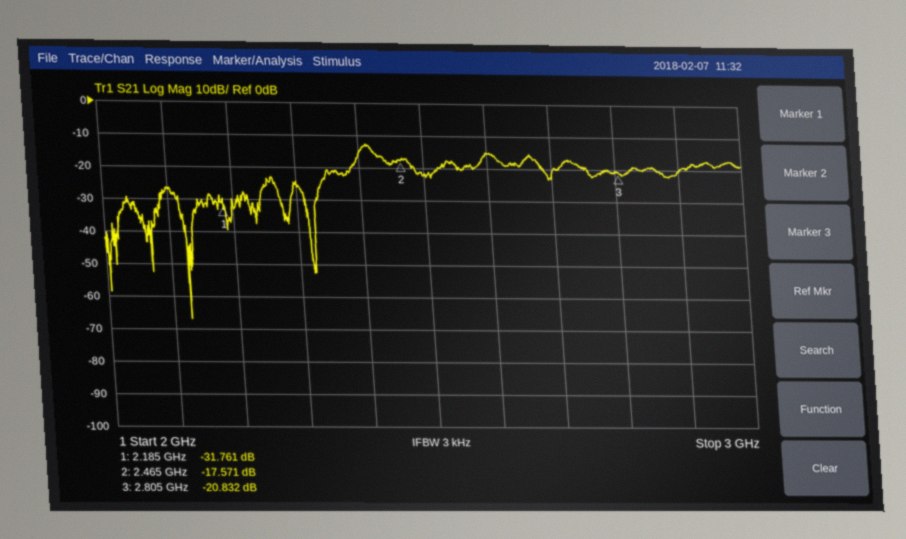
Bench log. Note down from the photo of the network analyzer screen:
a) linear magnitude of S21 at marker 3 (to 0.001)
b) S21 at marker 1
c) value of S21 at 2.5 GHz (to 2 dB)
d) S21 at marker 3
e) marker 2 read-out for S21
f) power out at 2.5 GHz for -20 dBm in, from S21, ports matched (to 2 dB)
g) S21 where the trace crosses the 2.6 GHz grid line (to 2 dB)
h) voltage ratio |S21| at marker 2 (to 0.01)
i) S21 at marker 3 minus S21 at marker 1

0.091
-31.761 dB
-22 dB
-20.832 dB
-17.571 dB
-42 dBm
-16 dB
0.13
10.929 dB
